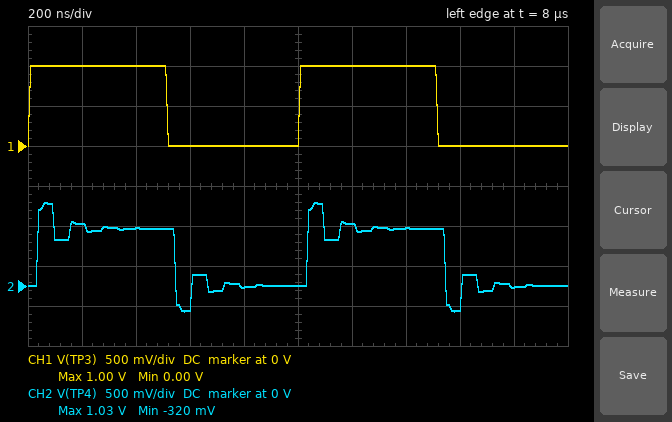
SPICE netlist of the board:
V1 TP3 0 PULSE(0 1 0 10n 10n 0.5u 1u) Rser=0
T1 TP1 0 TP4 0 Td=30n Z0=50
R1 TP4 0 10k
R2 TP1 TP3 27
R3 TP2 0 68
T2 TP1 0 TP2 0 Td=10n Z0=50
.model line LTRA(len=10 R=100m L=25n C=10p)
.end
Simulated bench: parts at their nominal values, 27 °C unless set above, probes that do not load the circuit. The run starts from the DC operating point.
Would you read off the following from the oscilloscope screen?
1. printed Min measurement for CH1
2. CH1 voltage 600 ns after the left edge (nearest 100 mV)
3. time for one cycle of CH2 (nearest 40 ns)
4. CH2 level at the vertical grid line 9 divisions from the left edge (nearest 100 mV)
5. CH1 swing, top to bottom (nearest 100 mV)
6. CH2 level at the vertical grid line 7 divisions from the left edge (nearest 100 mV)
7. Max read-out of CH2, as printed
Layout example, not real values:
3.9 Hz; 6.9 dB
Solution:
0.00 V; 0 V; 1.00 µs; 0 V; 1.0 V; 700 mV; 1.03 V
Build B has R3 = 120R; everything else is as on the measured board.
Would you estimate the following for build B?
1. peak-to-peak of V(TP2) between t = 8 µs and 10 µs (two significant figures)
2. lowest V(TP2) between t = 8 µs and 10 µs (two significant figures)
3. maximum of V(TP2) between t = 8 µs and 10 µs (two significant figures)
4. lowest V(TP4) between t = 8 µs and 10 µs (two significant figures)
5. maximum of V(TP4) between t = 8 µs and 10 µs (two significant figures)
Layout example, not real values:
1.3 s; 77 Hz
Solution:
1.0 V; -110 mV; 920 mV; -350 mV; 1.2 V
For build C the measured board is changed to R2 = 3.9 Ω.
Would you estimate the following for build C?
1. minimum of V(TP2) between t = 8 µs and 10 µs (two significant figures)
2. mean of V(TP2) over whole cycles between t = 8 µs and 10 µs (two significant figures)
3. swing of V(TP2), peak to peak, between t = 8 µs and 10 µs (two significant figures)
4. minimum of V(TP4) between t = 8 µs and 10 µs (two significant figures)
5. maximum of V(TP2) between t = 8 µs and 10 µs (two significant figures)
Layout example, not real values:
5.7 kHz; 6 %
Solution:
-71 mV; 480 mV; 1.1 V; -970 mV; 1.0 V
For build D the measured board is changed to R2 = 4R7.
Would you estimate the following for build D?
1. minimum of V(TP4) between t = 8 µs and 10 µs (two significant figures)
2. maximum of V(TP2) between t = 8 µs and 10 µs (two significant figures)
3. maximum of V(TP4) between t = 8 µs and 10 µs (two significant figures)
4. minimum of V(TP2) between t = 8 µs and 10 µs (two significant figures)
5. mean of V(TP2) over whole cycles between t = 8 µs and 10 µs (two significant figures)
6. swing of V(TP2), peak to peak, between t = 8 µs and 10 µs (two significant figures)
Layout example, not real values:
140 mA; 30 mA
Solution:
-900 mV; 1.0 V; 1.8 V; -76 mV; 480 mV; 1.1 V
